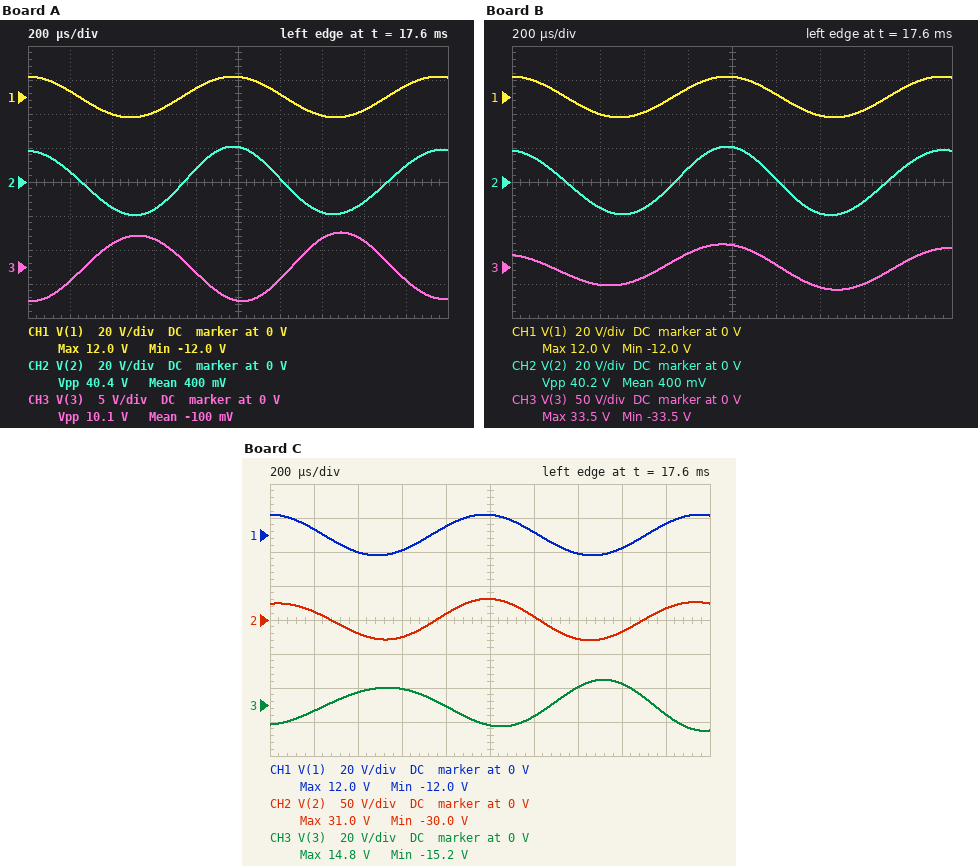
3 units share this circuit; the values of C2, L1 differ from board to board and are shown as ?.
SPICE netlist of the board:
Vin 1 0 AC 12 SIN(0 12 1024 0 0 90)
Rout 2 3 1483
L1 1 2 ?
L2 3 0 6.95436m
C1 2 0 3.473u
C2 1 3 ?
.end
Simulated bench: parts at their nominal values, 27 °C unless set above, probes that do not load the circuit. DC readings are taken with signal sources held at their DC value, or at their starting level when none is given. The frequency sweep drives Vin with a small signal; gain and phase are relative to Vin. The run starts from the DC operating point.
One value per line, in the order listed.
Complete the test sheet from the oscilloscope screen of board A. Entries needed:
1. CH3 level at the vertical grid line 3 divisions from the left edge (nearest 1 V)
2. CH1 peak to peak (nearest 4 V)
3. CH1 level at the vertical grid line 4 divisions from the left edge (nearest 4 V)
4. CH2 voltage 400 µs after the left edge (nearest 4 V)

4 V
24 V
4 V
-16 V
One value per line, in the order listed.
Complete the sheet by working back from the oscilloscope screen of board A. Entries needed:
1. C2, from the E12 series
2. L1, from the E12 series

1 µF
2.7 mH
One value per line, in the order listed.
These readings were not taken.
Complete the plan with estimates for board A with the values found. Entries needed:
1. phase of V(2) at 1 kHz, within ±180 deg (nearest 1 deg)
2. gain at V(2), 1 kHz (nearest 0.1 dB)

-1 deg
4.0 dB
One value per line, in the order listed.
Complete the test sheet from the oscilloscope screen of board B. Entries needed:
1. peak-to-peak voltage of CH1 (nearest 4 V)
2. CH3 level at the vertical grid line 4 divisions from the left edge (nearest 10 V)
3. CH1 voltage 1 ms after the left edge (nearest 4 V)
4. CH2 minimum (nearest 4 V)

24 V
20 V
12 V
-20 V
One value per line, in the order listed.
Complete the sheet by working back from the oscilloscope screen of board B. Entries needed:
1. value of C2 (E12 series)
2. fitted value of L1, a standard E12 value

6.8 µF
2.7 mH
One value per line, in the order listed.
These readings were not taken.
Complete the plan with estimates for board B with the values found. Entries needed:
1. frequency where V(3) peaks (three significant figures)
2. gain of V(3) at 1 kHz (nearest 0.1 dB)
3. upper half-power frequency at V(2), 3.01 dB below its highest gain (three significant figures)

732 Hz
6.7 dB
1.66 kHz
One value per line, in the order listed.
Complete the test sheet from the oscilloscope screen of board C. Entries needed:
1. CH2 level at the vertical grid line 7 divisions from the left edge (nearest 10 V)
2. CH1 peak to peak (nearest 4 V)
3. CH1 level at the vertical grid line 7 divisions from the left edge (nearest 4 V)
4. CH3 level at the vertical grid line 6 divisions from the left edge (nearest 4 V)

-30 V
24 V
-12 V
-8 V
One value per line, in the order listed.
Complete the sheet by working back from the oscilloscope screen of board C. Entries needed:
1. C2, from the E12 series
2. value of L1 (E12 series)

1.8 µF
3.9 mH
